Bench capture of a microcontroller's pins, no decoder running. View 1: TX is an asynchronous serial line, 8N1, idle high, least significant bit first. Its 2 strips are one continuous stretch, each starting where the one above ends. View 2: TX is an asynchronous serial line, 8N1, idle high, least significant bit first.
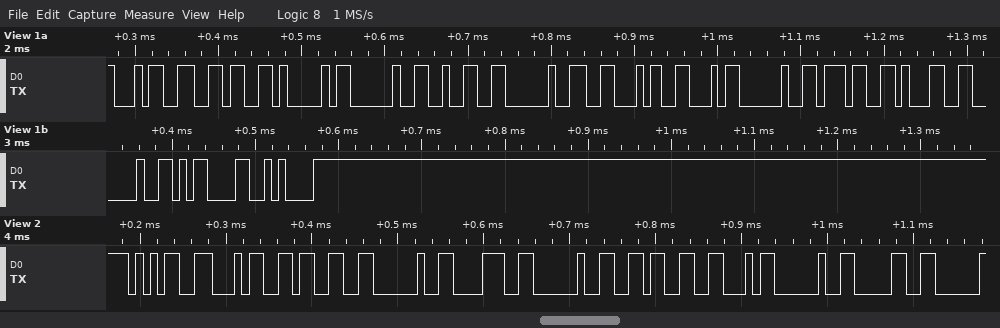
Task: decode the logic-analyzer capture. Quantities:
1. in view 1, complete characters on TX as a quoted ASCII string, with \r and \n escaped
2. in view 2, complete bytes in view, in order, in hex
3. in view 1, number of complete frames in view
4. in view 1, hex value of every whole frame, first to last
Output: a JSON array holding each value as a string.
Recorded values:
["\"46A 2 FF 71 \\r\\n\"", "35 34 33 20 38 20 36 46 20 30", "14", "34 36 41 20 32 20 46 46 20 37 31 20 0D 0A"]
